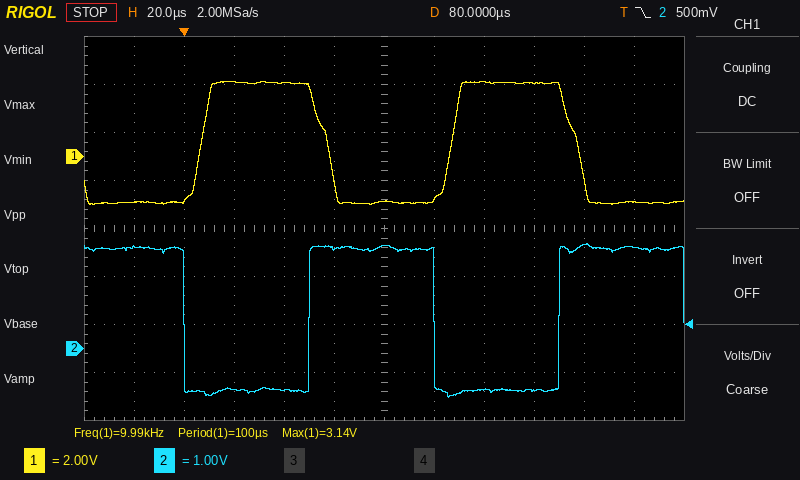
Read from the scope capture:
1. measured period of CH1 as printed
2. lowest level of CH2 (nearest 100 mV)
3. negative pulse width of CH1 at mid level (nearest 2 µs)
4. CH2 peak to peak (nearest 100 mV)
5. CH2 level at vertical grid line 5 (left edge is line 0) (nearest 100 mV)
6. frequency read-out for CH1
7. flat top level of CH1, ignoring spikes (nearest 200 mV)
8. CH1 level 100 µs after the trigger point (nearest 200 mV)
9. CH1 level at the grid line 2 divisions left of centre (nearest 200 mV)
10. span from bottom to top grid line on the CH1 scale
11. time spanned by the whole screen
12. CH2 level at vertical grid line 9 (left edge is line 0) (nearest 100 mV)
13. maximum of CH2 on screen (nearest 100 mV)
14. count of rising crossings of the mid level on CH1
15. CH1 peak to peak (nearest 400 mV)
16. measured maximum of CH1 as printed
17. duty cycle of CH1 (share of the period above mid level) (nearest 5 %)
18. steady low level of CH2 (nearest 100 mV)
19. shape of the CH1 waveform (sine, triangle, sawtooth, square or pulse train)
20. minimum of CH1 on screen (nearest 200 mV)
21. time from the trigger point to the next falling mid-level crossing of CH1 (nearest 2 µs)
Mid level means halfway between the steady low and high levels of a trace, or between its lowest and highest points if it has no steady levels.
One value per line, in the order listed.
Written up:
100 µs
-1.0 V
50 µs
3.2 V
2.1 V
9.99 kHz
3.0 V
-1.8 V
3.0 V
16 V
240 µs
-900 mV
2.2 V
2
5.2 V
3.14 V
50 %
-900 mV
square
-2.0 V
58 µs
